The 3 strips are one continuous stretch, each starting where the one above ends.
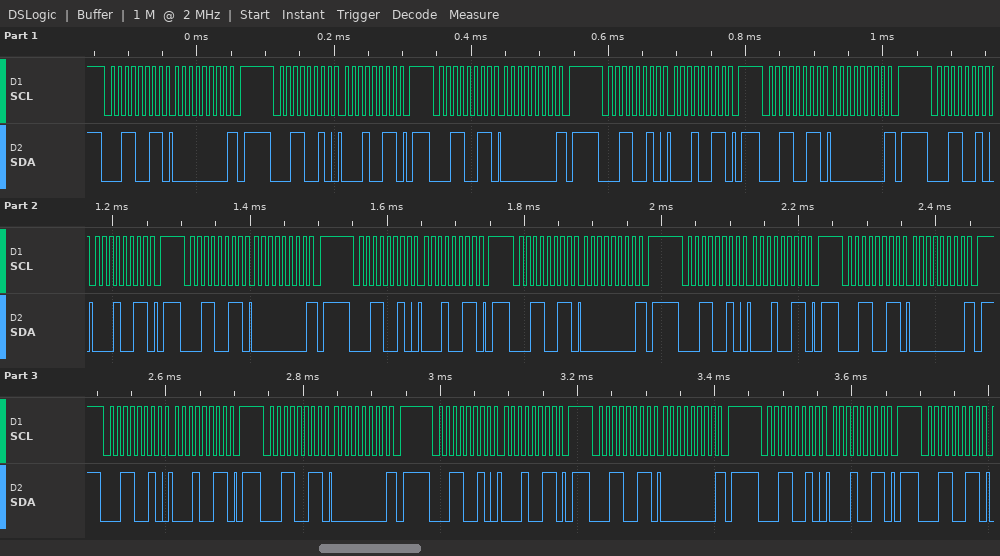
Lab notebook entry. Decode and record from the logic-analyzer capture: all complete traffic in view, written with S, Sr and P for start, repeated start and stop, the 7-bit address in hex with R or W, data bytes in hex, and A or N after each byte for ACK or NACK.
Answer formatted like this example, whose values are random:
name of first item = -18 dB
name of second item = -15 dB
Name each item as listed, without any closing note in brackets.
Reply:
all complete traffic in view, written with S, Sr and P for start, repeated start and stop, the 7-bit address in hex with R or W, data bytes in hex, and A or N after each byte for ACK or NACK = S 19R A 00 N P S 19W A 13 A P S 19R A 00 N P S 19W A 13 A P S 19R A 00 N P S 19W A 13 A P S 19R A 00 N P S 19W A 13 A P S 19R A 00 N P S 19W A 13 A P S 19R A 00 N P S 19W A 13 A P S 19R A 00 N P S 19W A 13 A P S 19R A 00 N P S 19W A 13 A P S 19R A
